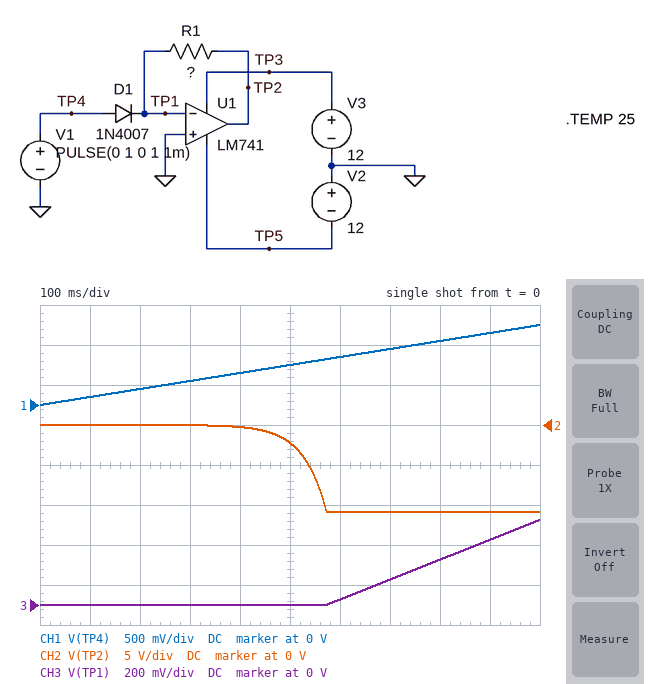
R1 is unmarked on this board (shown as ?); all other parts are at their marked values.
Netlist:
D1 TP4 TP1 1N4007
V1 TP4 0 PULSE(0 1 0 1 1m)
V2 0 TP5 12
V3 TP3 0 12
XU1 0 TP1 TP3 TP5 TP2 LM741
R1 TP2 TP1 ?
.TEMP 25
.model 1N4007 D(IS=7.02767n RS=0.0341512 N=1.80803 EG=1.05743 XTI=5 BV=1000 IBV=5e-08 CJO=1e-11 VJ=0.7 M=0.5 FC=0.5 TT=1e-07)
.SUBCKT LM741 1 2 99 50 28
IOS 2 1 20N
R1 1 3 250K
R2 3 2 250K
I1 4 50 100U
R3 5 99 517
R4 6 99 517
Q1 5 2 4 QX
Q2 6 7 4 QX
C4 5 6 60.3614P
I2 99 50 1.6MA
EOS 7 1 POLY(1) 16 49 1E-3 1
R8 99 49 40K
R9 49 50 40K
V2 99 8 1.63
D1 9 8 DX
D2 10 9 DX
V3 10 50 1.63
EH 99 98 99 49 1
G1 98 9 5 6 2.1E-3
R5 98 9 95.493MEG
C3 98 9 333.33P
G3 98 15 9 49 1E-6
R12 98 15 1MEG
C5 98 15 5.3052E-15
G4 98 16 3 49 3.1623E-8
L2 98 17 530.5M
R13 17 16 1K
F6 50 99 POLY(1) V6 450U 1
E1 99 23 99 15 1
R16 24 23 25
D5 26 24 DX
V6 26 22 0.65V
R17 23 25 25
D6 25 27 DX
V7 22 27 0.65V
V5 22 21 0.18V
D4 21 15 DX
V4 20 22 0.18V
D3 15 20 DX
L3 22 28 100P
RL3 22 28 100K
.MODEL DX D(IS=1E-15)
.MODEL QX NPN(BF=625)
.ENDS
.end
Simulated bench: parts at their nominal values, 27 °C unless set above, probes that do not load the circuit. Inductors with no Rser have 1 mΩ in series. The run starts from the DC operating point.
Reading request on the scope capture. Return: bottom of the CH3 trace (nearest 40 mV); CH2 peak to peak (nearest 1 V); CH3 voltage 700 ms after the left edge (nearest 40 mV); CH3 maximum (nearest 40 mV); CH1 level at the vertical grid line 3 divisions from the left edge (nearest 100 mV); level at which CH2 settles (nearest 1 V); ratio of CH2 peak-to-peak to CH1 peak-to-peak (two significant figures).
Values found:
0 V
11 V
120 mV
440 mV
300 mV
-11 V
11
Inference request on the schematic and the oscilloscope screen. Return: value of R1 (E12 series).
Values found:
8.2 kΩ
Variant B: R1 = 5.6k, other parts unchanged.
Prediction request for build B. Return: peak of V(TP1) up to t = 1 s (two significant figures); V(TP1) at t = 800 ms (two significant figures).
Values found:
410 mV
210 mV
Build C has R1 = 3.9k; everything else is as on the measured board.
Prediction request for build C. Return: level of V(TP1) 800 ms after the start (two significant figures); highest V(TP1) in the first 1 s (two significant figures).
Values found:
190 mV
390 mV
